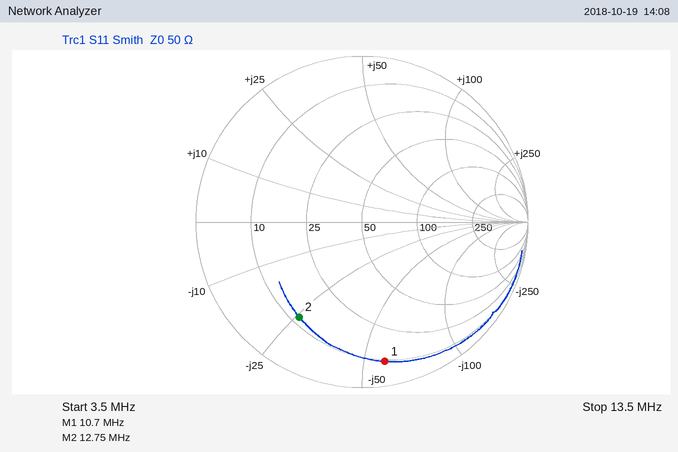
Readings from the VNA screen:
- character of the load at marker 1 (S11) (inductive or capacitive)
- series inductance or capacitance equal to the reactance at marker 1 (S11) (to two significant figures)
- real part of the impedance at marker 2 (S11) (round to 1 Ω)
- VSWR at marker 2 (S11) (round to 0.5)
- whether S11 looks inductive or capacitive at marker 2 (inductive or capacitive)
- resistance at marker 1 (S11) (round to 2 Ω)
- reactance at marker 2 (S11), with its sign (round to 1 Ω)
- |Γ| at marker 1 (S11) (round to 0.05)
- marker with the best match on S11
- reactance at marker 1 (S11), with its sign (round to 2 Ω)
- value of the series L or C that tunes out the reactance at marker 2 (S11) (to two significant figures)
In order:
capacitive
260 pF
12 Ω
5.5
capacitive
10 Ω
-26 Ω
0.85
marker 2
-58 Ω
320 nH
